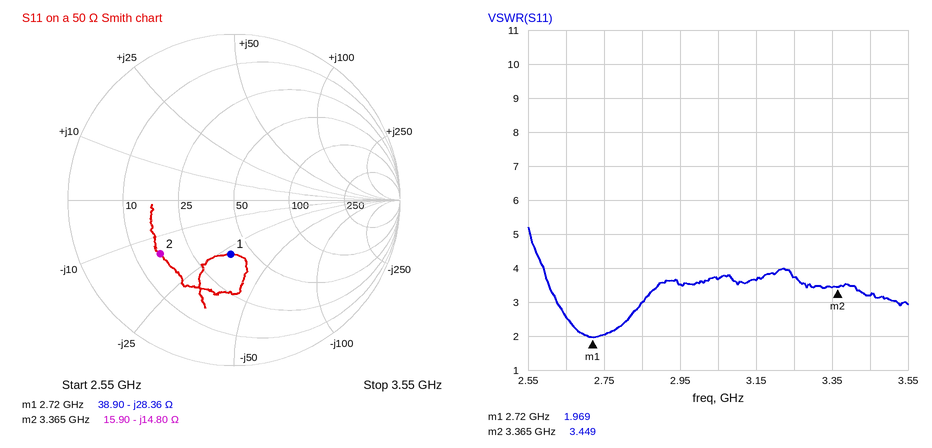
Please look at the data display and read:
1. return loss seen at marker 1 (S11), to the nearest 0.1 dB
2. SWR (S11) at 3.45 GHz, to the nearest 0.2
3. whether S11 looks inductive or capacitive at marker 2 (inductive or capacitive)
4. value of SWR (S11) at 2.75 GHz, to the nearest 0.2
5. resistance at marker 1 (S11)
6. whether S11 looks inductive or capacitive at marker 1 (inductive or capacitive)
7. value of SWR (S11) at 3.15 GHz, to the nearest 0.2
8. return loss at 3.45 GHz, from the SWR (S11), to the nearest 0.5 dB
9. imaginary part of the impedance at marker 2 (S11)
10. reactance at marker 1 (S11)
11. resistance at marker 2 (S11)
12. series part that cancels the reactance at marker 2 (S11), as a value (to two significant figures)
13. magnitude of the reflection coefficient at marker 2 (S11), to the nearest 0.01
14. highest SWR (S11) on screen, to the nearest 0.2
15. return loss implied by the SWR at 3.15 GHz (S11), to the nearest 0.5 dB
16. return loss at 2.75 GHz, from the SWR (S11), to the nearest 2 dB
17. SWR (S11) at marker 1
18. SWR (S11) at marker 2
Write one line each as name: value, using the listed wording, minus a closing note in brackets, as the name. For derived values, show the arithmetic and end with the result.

return loss seen at marker 1 (S11), to the nearest 0.1 dB: 9.7 dB
SWR (S11) at 3.45 GHz, to the nearest 0.2: 3.2
whether S11 looks inductive or capacitive at marker 2: capacitive
value of SWR (S11) at 2.75 GHz, to the nearest 0.2: 2.0
resistance at marker 1: 38.90 Ω
whether S11 looks inductive or capacitive at marker 1: capacitive
value of SWR (S11) at 3.15 GHz, to the nearest 0.2: 3.6
return loss at 3.45 GHz, from the SWR (S11), to the nearest 0.5 dB: −20 log10((3.2 − 1)/(3.2 + 1)) ≈ 5.62 dB, so 5.5 dB to the nearest 0.5 dB
imaginary part of the impedance at marker 2: -14.80 Ω
reactance at marker 1: -28.36 Ω
resistance at marker 2: 15.90 Ω
series part that cancels the reactance at marker 2 (S11), as a value: L = 14.8 Ω/(2π × 3.365 GHz) ≈ 700 pH
magnitude of the reflection coefficient at marker 2 (S11), to the nearest 0.01: 0.55
highest SWR (S11) on screen, to the nearest 0.2: 5.2
return loss implied by the SWR at 3.15 GHz (S11), to the nearest 0.5 dB: −20 log10((3.6 − 1)/(3.6 + 1)) ≈ 5.0 dB
return loss at 2.75 GHz, from the SWR (S11), to the nearest 2 dB: −20 log10((2 − 1)/(2 + 1)) ≈ 10 dB
SWR (S11) at marker 1: 1.969
SWR (S11) at marker 2: 3.449
